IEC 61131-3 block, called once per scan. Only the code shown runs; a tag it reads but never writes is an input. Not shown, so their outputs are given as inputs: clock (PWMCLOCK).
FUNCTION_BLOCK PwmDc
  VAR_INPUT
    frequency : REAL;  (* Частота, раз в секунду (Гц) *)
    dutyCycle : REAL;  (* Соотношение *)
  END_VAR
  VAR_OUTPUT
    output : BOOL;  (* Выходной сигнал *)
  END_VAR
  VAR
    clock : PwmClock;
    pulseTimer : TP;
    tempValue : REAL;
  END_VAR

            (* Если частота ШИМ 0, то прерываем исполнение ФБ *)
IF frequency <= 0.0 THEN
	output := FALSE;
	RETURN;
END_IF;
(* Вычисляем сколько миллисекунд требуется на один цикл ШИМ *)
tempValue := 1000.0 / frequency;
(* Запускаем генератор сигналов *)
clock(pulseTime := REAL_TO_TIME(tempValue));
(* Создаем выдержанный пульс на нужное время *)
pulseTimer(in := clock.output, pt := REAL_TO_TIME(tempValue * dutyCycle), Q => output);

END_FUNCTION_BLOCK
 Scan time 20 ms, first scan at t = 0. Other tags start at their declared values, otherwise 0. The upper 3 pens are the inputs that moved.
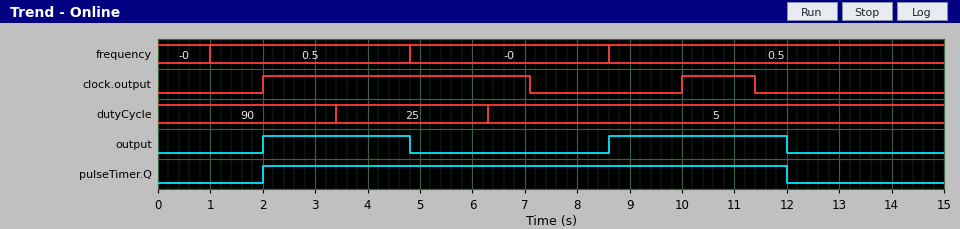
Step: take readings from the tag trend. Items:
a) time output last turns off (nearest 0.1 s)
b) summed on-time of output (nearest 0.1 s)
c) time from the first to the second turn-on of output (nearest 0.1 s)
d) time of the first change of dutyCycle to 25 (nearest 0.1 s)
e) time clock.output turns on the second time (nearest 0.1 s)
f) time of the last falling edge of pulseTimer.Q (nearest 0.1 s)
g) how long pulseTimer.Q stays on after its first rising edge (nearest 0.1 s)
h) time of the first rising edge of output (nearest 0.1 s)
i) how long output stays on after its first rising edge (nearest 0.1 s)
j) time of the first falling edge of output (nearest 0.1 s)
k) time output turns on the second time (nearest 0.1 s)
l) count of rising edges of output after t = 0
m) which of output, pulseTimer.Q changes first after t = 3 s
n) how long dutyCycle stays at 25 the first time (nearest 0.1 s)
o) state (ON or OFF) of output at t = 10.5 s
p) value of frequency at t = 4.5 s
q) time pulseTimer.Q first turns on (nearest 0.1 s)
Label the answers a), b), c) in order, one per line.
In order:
a) 12.0 s
b) 6.2 s
c) 6.6 s
d) 3.4 s
e) 10.0 s
f) 12.0 s
g) 10.0 s
h) 2.0 s
i) 2.8 s
j) 4.8 s
k) 8.6 s
l) 2
m) output
n) 2.9 s
o) ON
p) 0.5
q) 2.0 s
